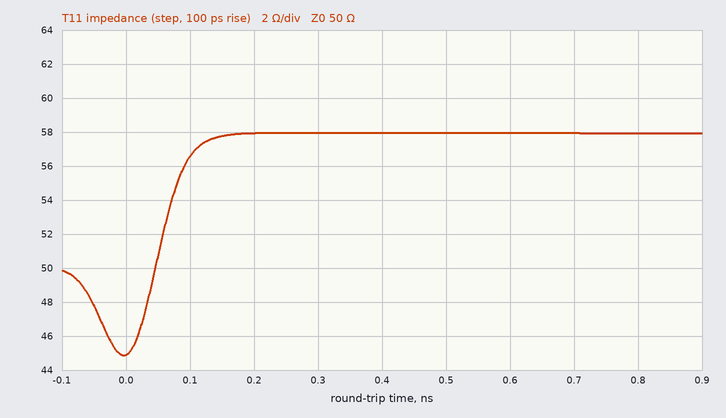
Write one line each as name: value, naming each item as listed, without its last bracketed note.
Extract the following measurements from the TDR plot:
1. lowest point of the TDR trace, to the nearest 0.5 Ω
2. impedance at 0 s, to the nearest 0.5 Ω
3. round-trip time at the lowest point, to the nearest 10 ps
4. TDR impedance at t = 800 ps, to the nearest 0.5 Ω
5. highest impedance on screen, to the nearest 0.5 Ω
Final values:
lowest point of the TDR trace, to the nearest 0.5 Ω: 45.0 Ω
impedance at 0 s, to the nearest 0.5 Ω: 45.0 Ω
round-trip time at the lowest point, to the nearest 10 ps: 0 ps
TDR impedance at t = 800 ps, to the nearest 0.5 Ω: 58.0 Ω
highest impedance on screen, to the nearest 0.5 Ω: 58.0 Ω
